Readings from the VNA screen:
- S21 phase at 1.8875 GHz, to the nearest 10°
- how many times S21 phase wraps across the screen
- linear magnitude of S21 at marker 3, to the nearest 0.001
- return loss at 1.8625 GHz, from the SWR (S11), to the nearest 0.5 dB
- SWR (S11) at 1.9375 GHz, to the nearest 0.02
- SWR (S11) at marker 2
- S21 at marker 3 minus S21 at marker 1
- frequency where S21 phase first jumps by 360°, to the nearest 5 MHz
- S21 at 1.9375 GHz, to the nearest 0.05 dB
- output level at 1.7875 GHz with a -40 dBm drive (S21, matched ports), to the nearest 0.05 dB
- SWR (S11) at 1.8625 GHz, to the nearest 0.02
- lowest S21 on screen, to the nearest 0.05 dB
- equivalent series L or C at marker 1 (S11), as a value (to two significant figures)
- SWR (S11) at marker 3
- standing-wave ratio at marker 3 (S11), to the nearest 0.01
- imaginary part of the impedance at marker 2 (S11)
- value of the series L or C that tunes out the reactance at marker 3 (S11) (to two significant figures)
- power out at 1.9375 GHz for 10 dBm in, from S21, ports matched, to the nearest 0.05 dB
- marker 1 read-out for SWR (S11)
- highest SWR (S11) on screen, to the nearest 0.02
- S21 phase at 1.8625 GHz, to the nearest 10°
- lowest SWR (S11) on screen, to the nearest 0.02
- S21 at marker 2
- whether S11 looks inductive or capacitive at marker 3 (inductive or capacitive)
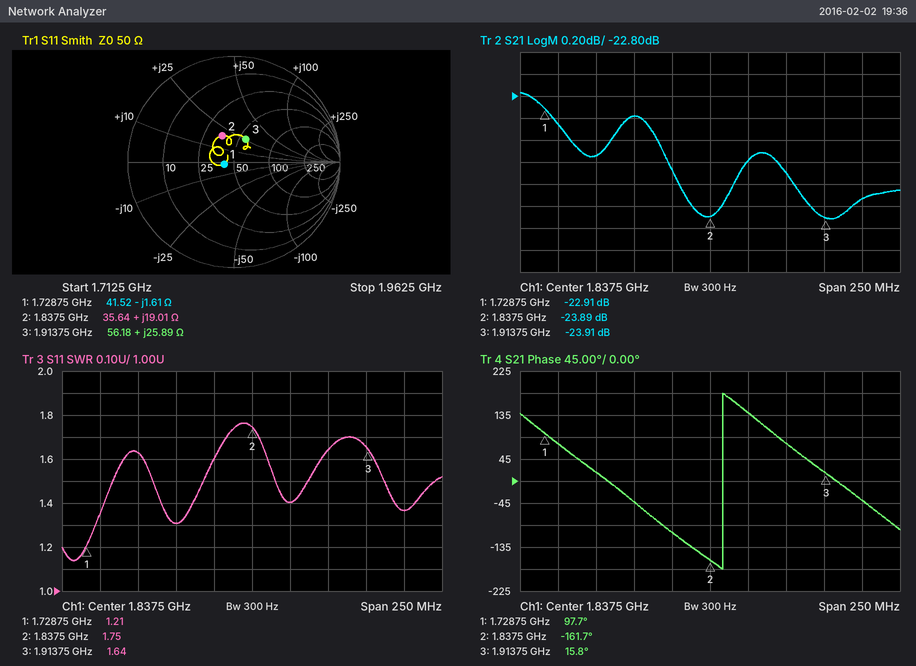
80°
1
0.064
15.5 dB
1.36
1.75
-1.00 dB
1.845 GHz
-23.75 dB
-63.00 dBm
1.40
-23.90 dB
57 pF
1.64
1.64
+19.01 Ω
3.2 pF
-13.75 dBm
1.21
1.76
140°
1.14
-23.89 dB
inductive
